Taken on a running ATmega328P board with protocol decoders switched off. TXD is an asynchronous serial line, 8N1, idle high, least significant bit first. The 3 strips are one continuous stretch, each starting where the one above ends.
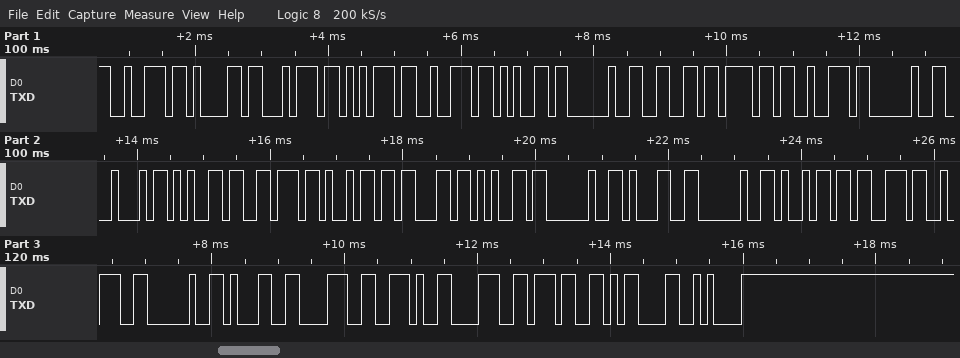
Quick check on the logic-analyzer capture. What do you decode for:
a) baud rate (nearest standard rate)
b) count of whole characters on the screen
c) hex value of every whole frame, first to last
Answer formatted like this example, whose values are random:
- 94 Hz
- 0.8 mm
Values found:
- 9600 baud
- 31
- 72 61 74 75 72 65 20 66 6F 72 20 44 65 76 69 63 65 20 31 20 69 73 3A 20 31 38 2E 38 37 0D 0A
